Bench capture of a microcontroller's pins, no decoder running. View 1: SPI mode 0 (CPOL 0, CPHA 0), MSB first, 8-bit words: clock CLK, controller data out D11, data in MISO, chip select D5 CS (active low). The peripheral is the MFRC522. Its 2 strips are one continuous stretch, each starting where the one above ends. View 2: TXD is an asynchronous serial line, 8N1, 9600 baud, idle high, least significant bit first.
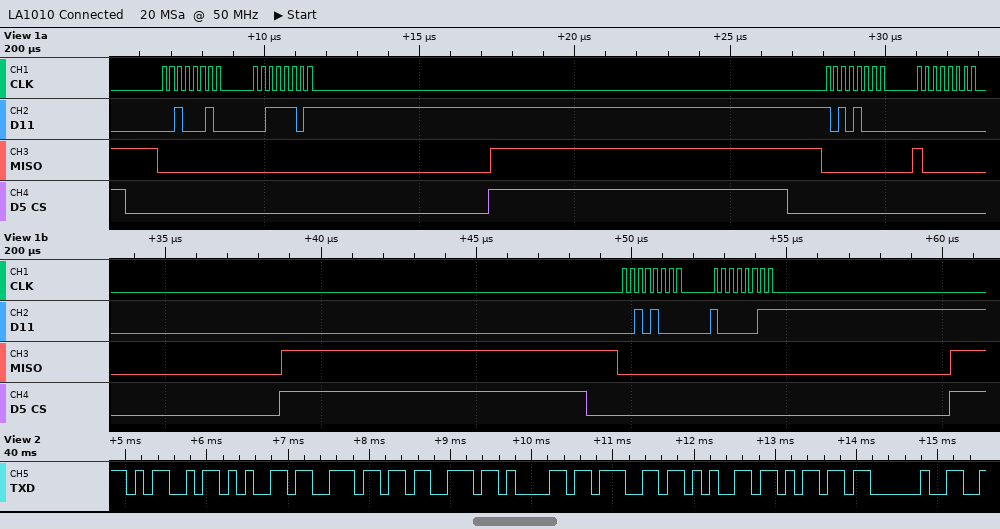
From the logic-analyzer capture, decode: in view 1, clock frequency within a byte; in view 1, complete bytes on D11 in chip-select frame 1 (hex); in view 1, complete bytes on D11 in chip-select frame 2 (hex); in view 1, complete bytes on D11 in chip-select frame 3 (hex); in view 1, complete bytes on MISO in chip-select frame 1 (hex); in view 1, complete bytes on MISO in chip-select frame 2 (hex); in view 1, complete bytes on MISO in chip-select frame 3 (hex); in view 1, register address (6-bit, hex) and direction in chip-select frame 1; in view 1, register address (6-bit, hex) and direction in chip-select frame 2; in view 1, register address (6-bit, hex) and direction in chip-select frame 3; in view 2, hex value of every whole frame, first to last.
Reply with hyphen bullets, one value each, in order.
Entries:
- 4 MHz
- 0x22 0x3D
- 0xA8 0x00
- 0x28 0x83
- 0x00 0x00
- 0x00 0x80
- 0x00 0x00
- 0x11 write
- 0x14 read
- 0x14 write
- 4D 65 6E 73 61 67 65 6D 20
